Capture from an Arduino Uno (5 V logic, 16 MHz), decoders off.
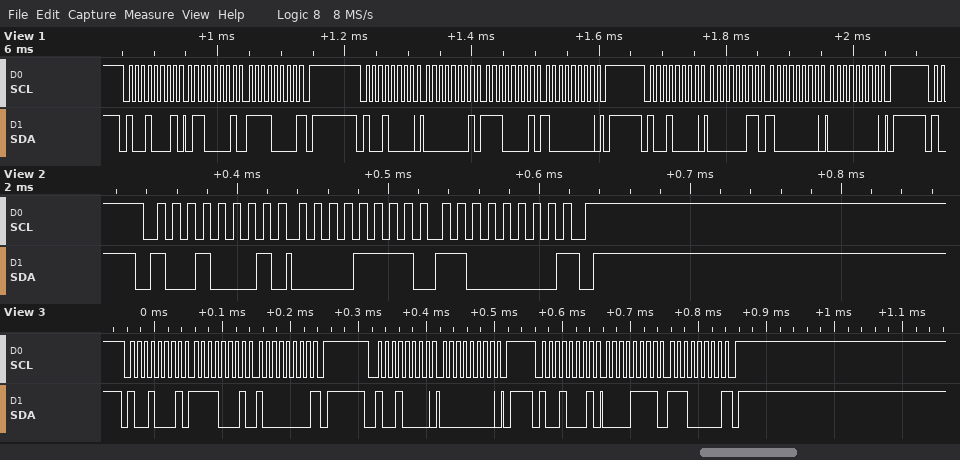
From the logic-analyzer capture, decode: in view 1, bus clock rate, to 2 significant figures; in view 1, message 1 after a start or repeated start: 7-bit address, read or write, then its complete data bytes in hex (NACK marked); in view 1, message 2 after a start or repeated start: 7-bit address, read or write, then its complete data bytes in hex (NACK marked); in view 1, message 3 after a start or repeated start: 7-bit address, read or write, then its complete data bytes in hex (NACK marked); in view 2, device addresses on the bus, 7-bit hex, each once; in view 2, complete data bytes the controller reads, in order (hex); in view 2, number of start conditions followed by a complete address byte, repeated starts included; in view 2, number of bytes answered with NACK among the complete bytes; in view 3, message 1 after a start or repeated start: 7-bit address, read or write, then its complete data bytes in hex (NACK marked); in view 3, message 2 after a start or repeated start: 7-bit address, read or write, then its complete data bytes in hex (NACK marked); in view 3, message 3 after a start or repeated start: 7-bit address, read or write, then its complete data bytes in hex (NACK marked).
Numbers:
100 kHz
0x48 read: 61 F0 NACK
0x48 write: 01 E1 80
0x48 write: 03 80 00
0x48
0F C0
1
1
0x48 read: F1 80 NACK
0x48 write: 00
0x48 read: 0F E0 NACK
